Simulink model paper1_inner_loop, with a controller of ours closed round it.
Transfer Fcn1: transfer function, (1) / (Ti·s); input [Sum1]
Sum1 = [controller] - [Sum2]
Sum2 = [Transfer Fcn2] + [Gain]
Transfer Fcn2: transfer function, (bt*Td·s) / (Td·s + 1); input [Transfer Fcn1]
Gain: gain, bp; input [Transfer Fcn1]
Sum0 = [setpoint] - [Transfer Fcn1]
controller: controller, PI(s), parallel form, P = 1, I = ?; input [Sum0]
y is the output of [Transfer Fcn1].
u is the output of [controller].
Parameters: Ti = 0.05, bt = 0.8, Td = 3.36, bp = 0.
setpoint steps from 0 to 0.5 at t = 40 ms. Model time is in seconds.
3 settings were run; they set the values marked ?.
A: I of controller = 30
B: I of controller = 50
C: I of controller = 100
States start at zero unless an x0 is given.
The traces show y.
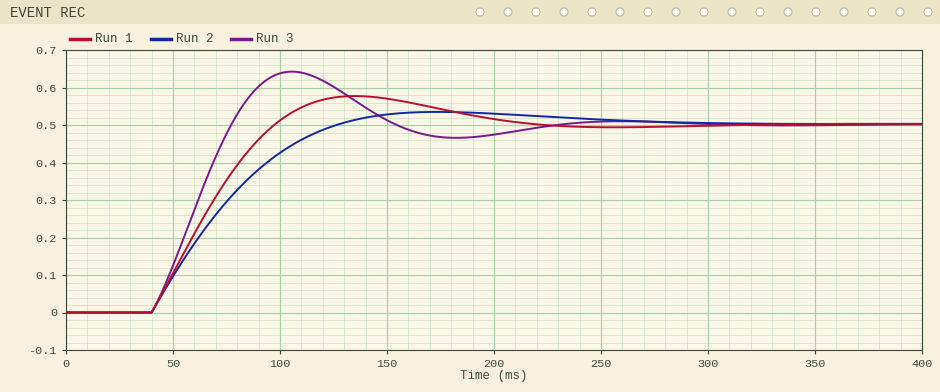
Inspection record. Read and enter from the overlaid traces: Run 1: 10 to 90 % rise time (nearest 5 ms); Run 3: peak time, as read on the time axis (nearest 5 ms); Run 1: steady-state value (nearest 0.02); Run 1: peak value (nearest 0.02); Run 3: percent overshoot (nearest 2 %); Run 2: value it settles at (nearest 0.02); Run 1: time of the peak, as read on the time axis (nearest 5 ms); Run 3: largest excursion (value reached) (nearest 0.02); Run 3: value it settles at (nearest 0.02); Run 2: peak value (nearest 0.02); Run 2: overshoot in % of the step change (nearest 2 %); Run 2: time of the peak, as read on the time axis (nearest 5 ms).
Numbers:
45 ms
105 ms
0.50
0.58
28 %
0.50
135 ms
0.64
0.50
0.54
6 %
175 ms
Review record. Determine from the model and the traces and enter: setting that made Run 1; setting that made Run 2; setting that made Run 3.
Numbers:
B
A
C
